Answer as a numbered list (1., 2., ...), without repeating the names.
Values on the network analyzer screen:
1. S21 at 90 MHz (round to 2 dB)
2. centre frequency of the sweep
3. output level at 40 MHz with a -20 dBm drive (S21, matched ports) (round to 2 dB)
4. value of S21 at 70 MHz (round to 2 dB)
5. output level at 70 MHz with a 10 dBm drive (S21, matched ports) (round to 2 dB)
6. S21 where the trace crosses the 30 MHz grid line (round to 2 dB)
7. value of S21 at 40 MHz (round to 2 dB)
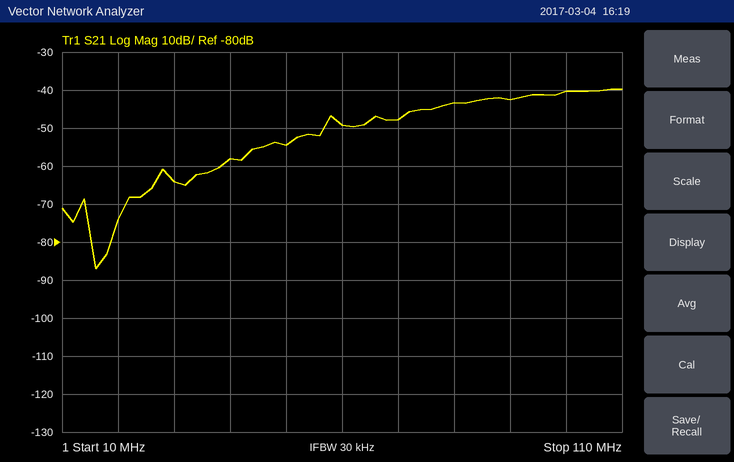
1. -42 dB
2. 60 MHz
3. -78 dBm
4. -48 dB
5. -38 dBm
6. -64 dB
7. -58 dB
